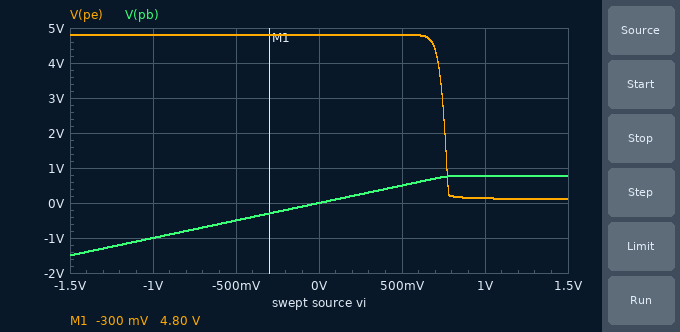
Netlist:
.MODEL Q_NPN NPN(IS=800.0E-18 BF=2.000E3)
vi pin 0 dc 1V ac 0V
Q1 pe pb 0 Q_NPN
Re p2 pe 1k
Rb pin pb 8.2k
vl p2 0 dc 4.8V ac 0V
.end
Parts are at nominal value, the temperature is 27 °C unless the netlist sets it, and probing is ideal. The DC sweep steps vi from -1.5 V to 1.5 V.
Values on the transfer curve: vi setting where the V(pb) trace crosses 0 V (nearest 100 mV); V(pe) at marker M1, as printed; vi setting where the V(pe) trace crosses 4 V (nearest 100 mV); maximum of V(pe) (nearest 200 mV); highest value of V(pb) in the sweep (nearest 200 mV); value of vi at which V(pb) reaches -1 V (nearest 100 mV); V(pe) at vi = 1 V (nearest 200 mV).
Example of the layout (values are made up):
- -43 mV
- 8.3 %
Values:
- 0 V
- 4.80 V
- 700 mV
- 4.8 V
- 800 mV
- -1.0 V
- 200 mV
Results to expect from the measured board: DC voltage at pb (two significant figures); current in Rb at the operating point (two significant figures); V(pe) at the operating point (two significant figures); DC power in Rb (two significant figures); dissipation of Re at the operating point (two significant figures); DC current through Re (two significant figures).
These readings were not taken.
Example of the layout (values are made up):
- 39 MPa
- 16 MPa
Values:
- 760 mV
- 29 µA
- 130 mV
- 7.0 µW
- 22 mW
- 4.7 mA
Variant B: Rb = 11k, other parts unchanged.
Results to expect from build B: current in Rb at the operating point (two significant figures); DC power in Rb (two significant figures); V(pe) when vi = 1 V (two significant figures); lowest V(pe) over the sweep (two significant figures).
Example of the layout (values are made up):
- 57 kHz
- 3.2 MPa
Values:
- 22 µA
- 5.2 µW
- 140 mV
- 110 mV
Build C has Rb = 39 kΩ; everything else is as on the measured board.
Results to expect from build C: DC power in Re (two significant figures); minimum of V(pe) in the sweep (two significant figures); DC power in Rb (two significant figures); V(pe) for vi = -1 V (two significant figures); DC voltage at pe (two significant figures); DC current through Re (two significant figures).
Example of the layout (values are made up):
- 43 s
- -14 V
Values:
- 21 mW
- 150 mV
- 1.5 µW
- 4.8 V
- 180 mV
- 4.6 mA
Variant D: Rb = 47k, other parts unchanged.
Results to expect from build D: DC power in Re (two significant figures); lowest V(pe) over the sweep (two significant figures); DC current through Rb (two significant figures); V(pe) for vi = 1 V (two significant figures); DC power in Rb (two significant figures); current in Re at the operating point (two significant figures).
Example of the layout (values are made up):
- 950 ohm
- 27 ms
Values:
- 21 mW
- 150 mV
- 5.1 µA
- 190 mV
- 1.2 µW
- 4.6 mA
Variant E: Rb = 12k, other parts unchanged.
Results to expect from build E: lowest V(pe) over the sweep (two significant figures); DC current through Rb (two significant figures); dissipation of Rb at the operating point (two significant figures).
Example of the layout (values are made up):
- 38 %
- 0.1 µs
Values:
- 110 mV
- 20 µA
- 4.8 µW
